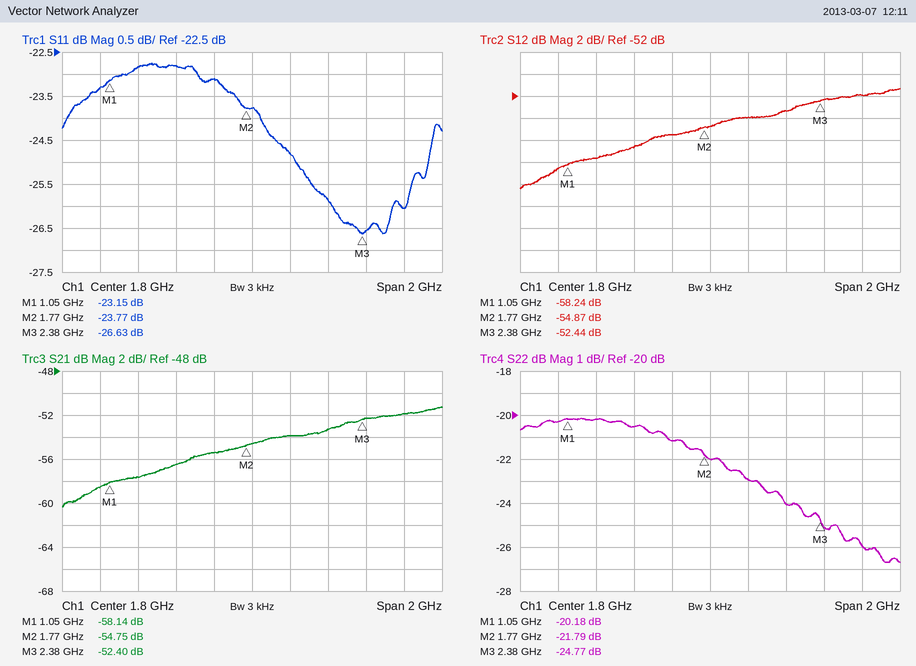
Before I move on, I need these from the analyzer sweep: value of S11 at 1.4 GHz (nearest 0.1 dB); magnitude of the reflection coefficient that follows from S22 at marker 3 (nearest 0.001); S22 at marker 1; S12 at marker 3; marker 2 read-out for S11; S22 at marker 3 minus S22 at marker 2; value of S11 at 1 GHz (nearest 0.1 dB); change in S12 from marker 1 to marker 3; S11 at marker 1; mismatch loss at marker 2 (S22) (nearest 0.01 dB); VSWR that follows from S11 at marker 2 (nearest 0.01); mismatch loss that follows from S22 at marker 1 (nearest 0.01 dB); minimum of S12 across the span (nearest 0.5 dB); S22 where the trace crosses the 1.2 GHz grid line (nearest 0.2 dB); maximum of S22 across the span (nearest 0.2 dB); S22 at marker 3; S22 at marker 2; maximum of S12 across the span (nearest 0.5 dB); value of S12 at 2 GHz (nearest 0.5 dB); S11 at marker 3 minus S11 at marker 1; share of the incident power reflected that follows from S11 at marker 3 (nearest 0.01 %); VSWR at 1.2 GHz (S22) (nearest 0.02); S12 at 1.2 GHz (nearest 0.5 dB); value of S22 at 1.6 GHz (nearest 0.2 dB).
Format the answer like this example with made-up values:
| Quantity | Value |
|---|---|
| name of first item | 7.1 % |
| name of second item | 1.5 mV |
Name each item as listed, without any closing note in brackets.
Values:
| Quantity | Value |
|---|---|
| value of S11 at 1.4 GHz | -22.8 dB |
| magnitude of the reflection coefficient that follows from S22 at marker 3 | 0.058 |
| S22 at marker 1 | -20.18 dB |
| S12 at marker 3 | -52.44 dB |
| marker 2 read-out for S11 | -23.77 dB |
| S22 at marker 3 minus S22 at marker 2 | -2.98 dB |
| value of S11 at 1 GHz | -23.3 dB |
| change in S12 from marker 1 to marker 3 | 5.80 dB |
| S11 at marker 1 | -23.15 dB |
| mismatch loss at marker 2 (S22) | 0.03 dB |
| VSWR that follows from S11 at marker 2 | 1.14 |
| mismatch loss that follows from S22 at marker 1 | 0.04 dB |
| minimum of S12 across the span | -60.5 dB |
| S22 where the trace crosses the 1.2 GHz grid line | -20.2 dB |
| maximum of S22 across the span | -20.2 dB |
| S22 at marker 3 | -24.77 dB |
| S22 at marker 2 | -21.79 dB |
| maximum of S12 across the span | -51.5 dB |
| value of S12 at 2 GHz | -54.0 dB |
| S11 at marker 3 minus S11 at marker 1 | -3.48 dB |
| share of the incident power reflected that follows from S11 at marker 3 | 0.22 % |
| VSWR at 1.2 GHz (S22) | 1.22 |
| S12 at 1.2 GHz | -57.5 dB |
| value of S22 at 1.6 GHz | -21.2 dB |
